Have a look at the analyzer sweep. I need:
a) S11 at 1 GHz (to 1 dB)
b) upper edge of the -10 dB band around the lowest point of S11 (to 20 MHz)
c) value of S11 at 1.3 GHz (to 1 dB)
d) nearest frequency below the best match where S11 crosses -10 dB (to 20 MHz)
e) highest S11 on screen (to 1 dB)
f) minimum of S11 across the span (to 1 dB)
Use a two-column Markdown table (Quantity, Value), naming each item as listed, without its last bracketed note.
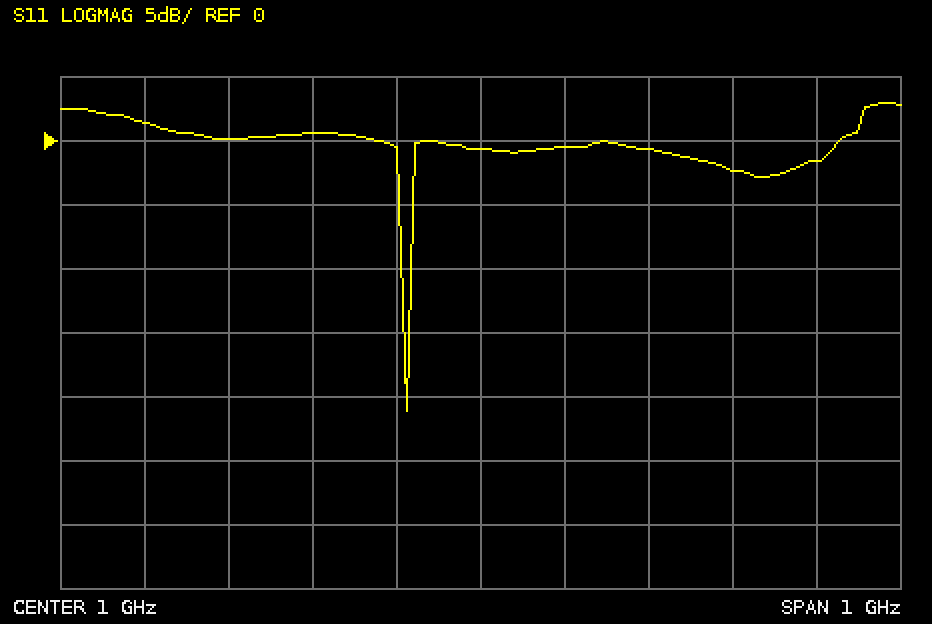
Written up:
| Quantity | Value |
|---|---|
| S11 at 1 GHz | -1 dB |
| upper edge of the -10 dB band around the lowest point of S11 | 920 MHz |
| value of S11 at 1.3 GHz | -2 dB |
| nearest frequency below the best match where S11 crosses -10 dB | 900 MHz |
| highest S11 on screen | 3 dB |
| minimum of S11 across the span | -21 dB |
